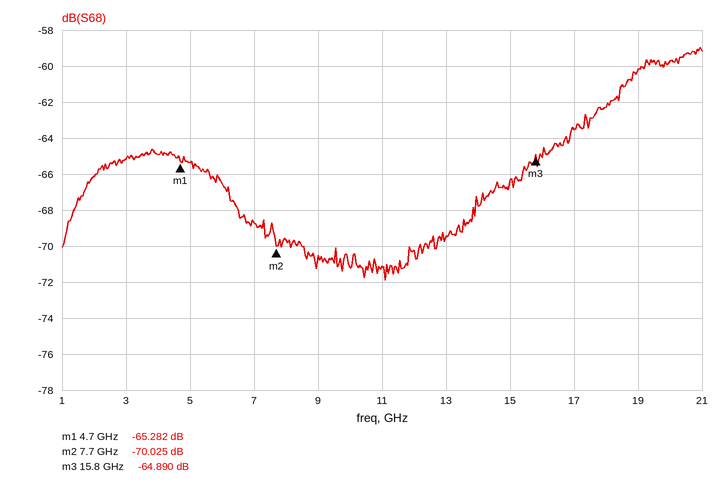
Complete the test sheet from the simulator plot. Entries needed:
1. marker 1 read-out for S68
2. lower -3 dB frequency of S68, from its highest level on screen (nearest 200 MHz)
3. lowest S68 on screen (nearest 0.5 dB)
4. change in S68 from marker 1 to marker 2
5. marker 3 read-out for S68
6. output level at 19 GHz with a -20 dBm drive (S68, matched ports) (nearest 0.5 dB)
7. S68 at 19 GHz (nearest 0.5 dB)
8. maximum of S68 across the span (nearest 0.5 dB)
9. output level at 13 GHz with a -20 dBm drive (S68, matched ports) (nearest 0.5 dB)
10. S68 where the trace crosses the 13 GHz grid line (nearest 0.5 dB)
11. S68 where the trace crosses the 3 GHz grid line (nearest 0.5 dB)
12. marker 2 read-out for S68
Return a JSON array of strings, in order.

["-65.282 dB", "18.2 GHz", "-72.0 dB", "-4.743 dB", "-64.890 dB", "-80.0 dBm", "-60.0 dB", "-59.0 dB", "-89.5 dBm", "-69.5 dB", "-65.0 dB", "-70.025 dB"]
